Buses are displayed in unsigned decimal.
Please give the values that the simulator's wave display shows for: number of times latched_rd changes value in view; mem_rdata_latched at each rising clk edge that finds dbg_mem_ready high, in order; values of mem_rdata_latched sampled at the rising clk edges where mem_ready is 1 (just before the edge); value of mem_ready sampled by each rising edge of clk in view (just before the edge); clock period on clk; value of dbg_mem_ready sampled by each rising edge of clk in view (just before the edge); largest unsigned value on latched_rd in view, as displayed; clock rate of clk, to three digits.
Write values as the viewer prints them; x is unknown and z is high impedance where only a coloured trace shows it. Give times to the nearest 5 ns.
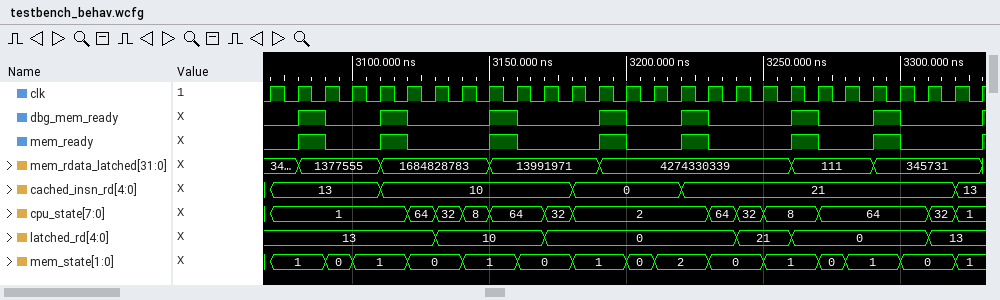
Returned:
5
1377555, 1684828783, 13991971, 4274330339, 4274330339, 111, 345731
1377555, 1684828783, 13991971, 4274330339, 4274330339, 111, 345731
0 0 1 0 0 1 0 0 0 1 0 0 0 1 0 0 1 0 0 0 1 0 0 1 0 0 0
10 ns
0 0 1 0 0 1 0 0 0 1 0 0 0 1 0 0 1 0 0 0 1 0 0 1 0 0 0
21
100 MHz
